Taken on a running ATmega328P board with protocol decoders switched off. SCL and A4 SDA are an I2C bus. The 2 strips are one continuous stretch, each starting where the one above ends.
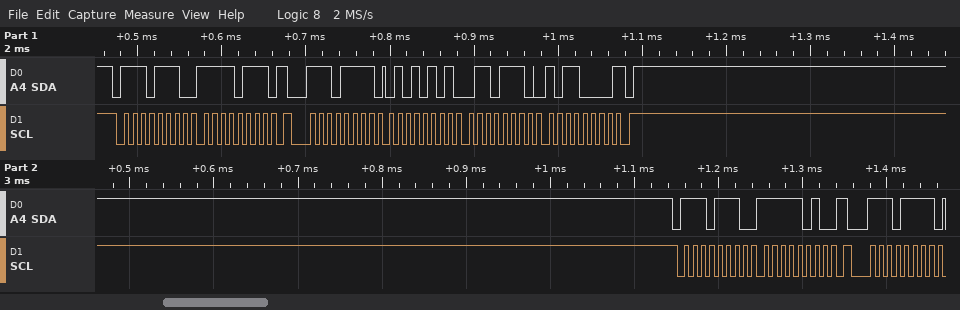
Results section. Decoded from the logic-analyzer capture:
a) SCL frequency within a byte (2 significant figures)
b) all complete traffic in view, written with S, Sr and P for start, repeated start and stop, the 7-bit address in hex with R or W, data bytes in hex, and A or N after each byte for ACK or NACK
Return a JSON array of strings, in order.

["100 kHz", "S 77W A F7 A Sr 77R A 55 A 6E A B0 N P S 77W A FA A Sr 77R A"]
